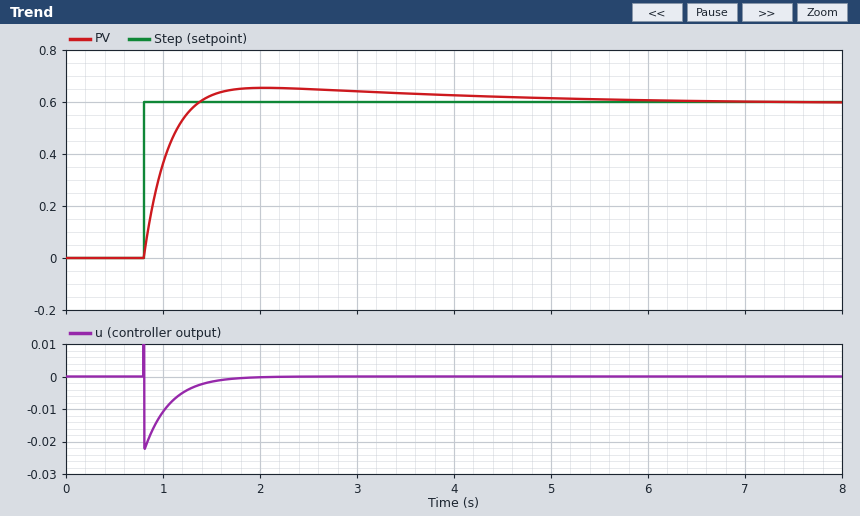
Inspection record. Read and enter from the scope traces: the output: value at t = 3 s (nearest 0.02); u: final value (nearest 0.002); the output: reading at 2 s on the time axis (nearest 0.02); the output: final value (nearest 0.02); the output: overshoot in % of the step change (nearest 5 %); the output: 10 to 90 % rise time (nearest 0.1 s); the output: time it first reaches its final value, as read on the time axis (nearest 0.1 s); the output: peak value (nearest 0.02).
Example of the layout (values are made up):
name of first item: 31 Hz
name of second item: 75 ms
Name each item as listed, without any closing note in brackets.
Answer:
the output: value at t = 3 s: 0.64
u: final value: 0.000
the output: reading at 2 s on the time axis: 0.66
the output: final value: 0.60
the output: overshoot in % of the step change: 10 %
the output: 10 to 90 % rise time: 0.4 s
the output: time it first reaches its final value, as read on the time axis: 1.4 s
the output: peak value: 0.66
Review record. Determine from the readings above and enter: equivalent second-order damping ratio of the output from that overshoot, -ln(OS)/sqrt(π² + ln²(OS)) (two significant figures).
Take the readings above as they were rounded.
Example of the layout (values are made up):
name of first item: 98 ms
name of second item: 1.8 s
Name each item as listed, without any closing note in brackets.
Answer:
equivalent second-order damping ratio of the output from that overshoot, -ln(OS)/sqrt(π² + ln²(OS)): 0.59
